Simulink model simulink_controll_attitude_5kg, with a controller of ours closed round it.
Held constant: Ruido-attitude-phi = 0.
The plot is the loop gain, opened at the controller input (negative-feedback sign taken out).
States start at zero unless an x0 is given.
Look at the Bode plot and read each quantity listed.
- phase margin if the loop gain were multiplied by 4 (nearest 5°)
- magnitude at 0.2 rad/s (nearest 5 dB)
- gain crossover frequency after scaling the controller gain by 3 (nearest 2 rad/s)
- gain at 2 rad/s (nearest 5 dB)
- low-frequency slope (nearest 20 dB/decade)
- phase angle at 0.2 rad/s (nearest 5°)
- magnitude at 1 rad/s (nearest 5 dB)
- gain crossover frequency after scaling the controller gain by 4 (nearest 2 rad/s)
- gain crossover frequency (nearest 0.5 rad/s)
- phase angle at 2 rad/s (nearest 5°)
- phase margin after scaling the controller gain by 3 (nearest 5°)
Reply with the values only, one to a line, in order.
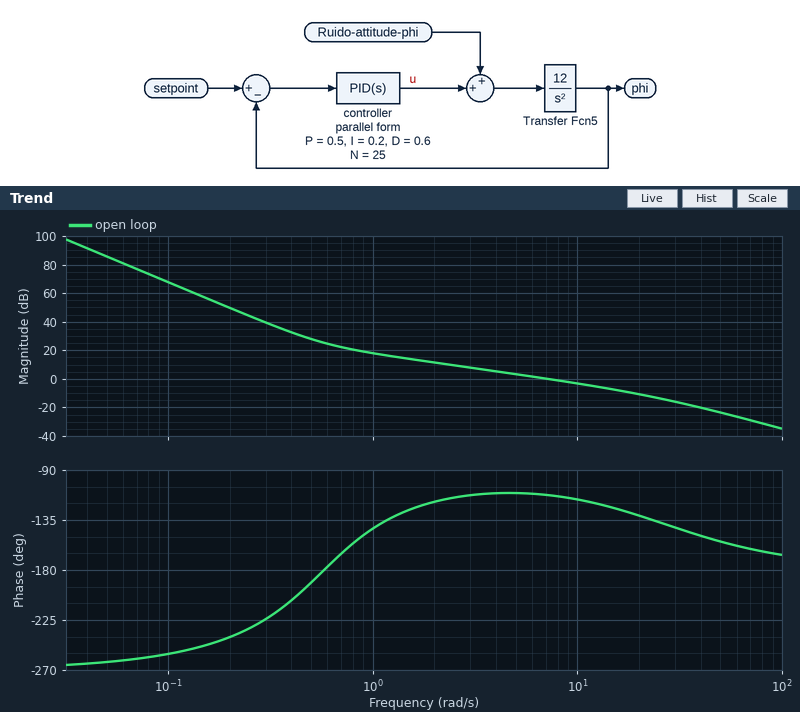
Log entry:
45°
50 dB
18 rad/s
10 dB
-60 dB/decade
-240°
20 dB
22 rad/s
7.0 rad/s
-120°
50°
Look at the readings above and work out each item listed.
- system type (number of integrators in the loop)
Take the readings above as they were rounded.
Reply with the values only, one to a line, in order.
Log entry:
3
